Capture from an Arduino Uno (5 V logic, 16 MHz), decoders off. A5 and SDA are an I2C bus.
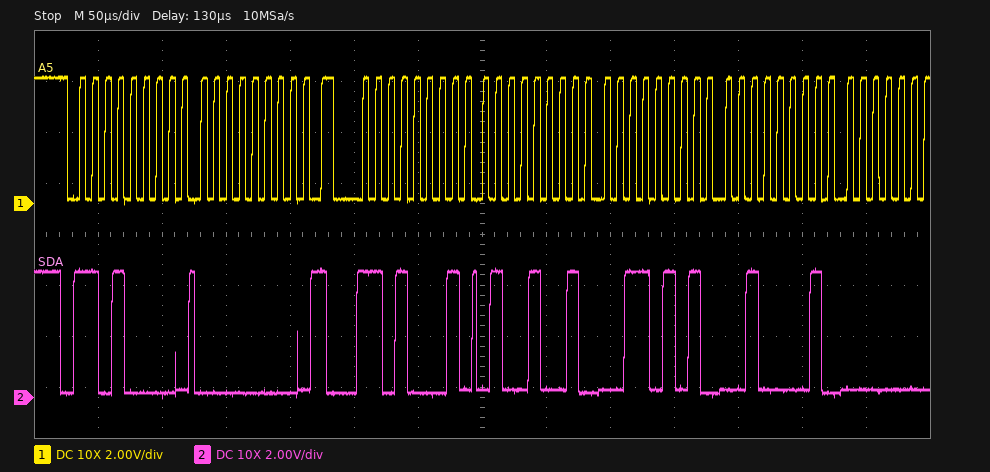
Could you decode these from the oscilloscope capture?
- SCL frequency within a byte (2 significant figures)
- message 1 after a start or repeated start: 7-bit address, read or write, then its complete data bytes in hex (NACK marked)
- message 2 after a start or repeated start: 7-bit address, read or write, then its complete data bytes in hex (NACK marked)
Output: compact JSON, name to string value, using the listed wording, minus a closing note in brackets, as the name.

{"SCL frequency within a byte": "100 kHz", "message 1 after a start or repeated start: 7-bit address, read or write, then its complete data bytes in hex": "0x68 write: 00", "message 2 after a start or repeated start: 7-bit address, read or write, then its complete data bytes in hex": "0x68 read: 49 35 21"}
